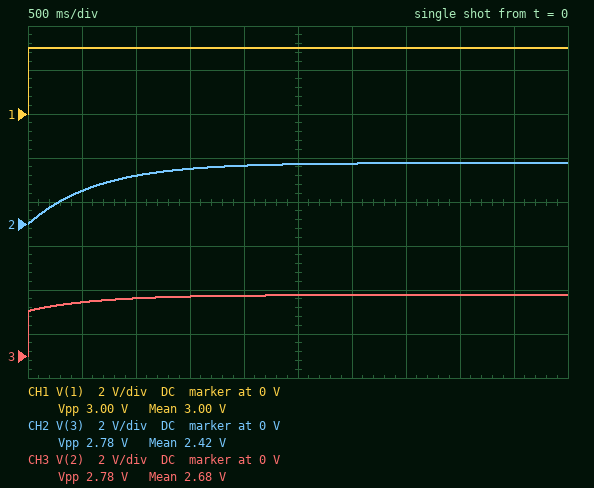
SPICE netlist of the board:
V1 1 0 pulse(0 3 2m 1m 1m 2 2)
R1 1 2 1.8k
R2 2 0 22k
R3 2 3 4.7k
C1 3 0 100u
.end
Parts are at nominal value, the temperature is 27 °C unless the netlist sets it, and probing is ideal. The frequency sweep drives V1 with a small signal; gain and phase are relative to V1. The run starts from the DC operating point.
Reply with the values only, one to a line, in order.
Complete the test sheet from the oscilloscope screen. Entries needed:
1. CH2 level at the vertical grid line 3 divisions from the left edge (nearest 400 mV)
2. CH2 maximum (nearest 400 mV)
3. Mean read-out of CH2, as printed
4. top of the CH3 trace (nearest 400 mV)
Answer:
2.4 V
2.8 V
2.42 V
2.8 V
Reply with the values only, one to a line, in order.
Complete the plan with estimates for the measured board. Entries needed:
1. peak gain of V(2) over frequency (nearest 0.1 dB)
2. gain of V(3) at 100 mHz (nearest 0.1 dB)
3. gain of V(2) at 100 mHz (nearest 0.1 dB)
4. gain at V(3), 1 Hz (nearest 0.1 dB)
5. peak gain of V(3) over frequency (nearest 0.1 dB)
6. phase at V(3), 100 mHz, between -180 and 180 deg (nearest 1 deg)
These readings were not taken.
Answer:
-0.7 dB
-1.3 dB
-1.0 dB
-13.0 dB
-0.7 dB
-22 deg
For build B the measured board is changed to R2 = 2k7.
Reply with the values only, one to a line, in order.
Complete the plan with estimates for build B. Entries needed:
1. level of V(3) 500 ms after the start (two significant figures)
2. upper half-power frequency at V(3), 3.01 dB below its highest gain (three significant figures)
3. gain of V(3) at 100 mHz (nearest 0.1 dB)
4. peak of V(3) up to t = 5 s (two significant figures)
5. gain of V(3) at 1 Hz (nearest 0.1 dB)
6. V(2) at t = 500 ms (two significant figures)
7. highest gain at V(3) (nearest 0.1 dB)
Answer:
1.0 V
275 mHz
-5.0 dB
1.8 V
-16.0 dB
1.7 V
-4.4 dB
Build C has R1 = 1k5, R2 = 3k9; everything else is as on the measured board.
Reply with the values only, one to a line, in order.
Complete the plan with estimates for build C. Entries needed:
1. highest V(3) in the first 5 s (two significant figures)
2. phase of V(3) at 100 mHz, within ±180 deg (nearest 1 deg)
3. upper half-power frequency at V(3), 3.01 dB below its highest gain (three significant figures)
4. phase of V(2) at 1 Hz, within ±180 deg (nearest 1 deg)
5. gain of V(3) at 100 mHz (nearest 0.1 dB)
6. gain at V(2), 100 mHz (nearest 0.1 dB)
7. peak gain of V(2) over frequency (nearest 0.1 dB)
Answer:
2.2 V
-20 deg
275 mHz
-3 deg
-3.4 dB
-3.0 dB
-2.8 dB
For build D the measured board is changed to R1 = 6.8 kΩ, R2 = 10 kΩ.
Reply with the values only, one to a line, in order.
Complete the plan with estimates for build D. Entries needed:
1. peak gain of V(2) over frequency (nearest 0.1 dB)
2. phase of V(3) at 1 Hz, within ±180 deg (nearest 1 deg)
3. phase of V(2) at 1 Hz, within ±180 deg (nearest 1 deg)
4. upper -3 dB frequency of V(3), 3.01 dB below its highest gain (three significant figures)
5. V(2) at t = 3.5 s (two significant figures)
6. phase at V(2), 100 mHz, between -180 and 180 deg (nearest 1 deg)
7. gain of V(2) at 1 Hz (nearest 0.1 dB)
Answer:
-4.5 dB
-80 deg
-8 deg
182 mHz
1.8 V
-12 deg
-9.6 dB
